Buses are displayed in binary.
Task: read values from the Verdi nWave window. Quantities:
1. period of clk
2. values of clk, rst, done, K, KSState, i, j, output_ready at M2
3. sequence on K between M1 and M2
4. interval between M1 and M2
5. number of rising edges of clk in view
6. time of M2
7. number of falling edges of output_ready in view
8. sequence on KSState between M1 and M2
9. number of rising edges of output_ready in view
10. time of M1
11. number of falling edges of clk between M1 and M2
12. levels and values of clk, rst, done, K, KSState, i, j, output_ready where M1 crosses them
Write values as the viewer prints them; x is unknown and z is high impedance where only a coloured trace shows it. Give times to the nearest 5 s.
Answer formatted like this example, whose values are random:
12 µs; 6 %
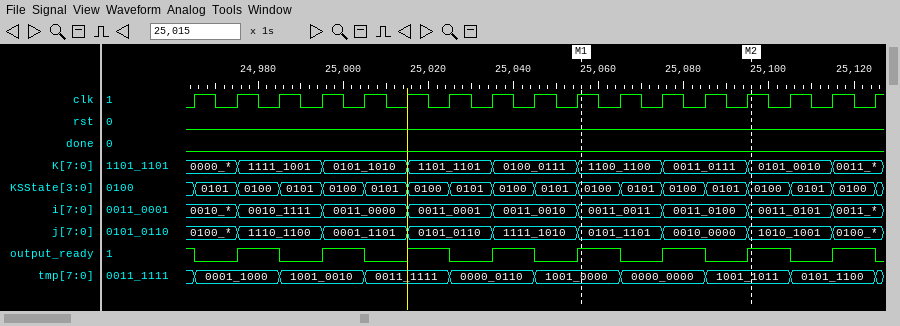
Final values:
10 s; clk=1, rst=0, done=0, K=0101_0010, KSState=0100, i=0011_0101, j=1010_1001, output_ready=1; 1100_1100, 0011_0111, 0101_0010; 40 s; 17; 25095 s; 9; 0100, 0101, 0100, 0101, 0100; 8; 25055 s; 4; clk=1, rst=0, done=0, K=1100_1100, KSState=0100, i=0011_0011, j=0101_1101, output_ready=1
